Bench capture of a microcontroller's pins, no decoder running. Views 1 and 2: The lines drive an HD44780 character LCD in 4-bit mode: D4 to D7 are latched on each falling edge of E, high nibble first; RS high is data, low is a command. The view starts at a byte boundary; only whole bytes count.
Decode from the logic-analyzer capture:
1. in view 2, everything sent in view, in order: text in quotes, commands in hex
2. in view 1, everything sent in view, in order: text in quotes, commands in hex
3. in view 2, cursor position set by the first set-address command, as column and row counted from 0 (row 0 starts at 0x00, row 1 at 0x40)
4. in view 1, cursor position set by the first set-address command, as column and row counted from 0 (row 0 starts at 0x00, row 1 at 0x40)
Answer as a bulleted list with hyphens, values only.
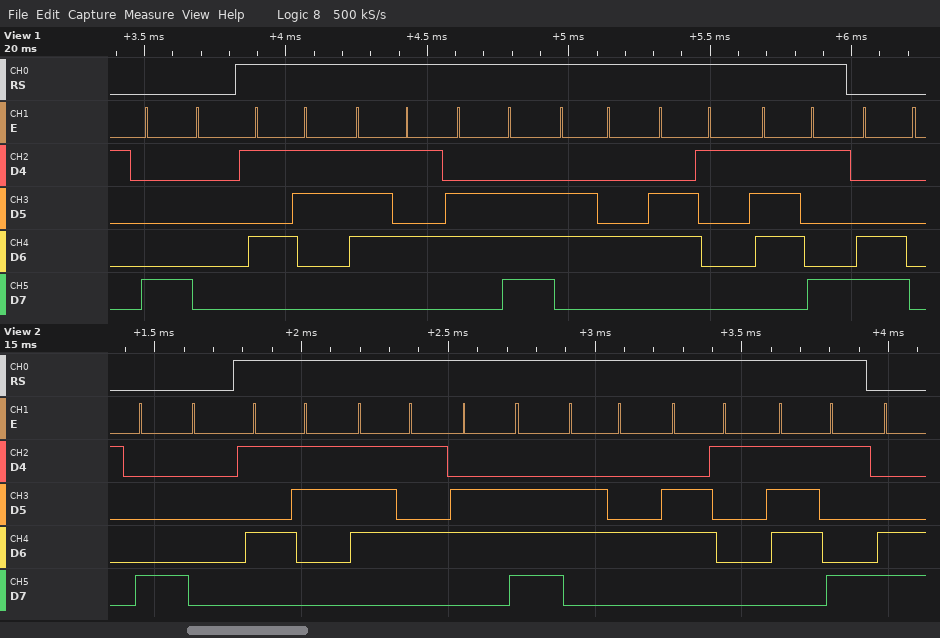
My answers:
- 0x80 "Sunday"
- 0x80 "Sunday" 0xC0
- column 0, row 0
- column 0, row 0
